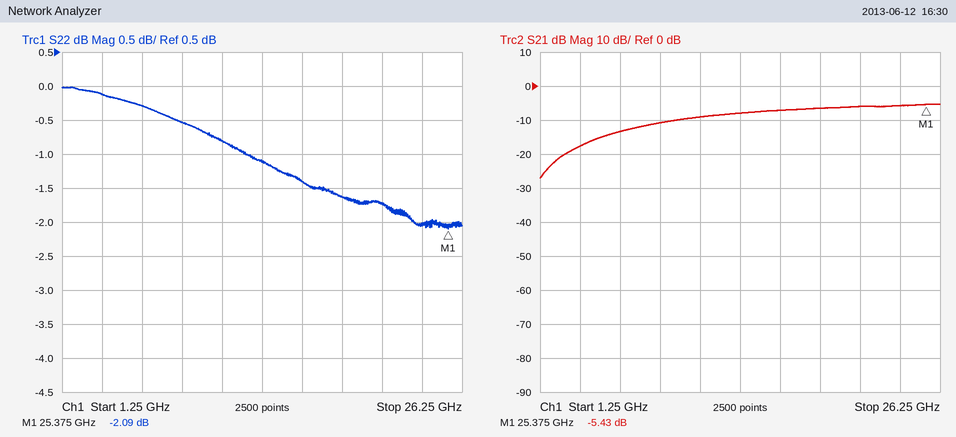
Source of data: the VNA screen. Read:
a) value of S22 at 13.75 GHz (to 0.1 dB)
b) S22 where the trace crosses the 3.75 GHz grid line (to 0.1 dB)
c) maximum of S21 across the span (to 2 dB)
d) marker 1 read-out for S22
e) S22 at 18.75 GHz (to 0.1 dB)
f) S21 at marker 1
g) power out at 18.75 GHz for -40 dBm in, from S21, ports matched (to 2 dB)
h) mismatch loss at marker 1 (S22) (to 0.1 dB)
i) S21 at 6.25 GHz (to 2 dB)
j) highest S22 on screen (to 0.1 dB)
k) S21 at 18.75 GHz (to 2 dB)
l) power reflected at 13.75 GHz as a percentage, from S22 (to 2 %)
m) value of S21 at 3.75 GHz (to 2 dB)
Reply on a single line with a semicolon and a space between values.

-1.1 dB; -0.1 dB; -6 dB; -2.09 dB; -1.6 dB; -5.43 dB; -46 dBm; 4.2 dB; -14 dB; 0.0 dB; -6 dB; 78 %; -18 dB
